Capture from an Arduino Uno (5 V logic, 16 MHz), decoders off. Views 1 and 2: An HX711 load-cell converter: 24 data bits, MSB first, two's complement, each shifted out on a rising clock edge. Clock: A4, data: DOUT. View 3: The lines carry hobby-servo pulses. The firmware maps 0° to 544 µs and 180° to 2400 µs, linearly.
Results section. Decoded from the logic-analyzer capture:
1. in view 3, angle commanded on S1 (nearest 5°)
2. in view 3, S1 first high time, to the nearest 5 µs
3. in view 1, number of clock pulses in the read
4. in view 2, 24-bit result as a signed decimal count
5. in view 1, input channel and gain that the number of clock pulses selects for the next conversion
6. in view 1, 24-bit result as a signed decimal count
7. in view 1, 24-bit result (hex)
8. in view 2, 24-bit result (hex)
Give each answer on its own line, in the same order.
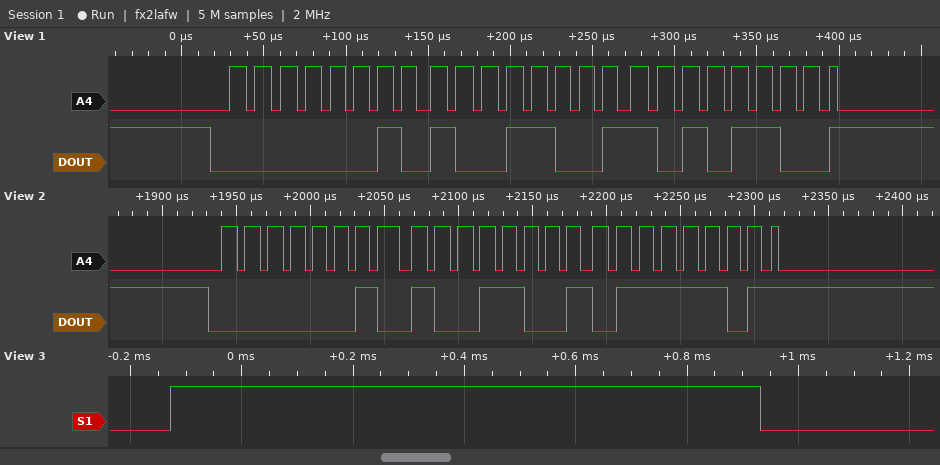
50°
1060 µs
25
170365
channel A, gain 128
170412
0x0299AC
0x02997D
